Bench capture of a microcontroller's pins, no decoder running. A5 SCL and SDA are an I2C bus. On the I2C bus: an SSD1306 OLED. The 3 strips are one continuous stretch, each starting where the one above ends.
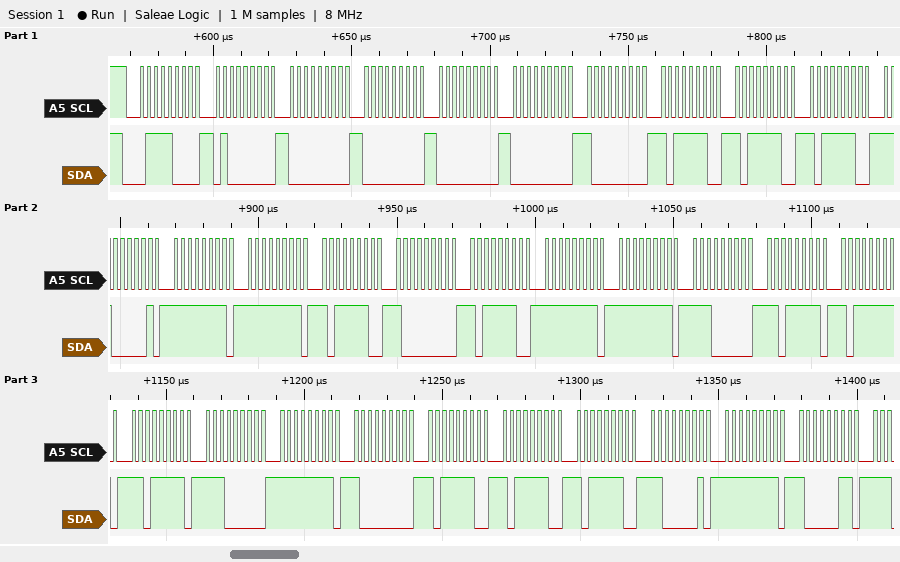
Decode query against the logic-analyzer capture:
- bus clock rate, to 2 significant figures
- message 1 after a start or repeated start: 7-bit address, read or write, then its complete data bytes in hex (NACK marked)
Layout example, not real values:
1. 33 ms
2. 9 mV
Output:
1. 400 kHz
2. 0x3C write: 40 00 00 00 00 80 BE BE BE C1 FF FF BE 80 BE FF FF E0 DF BF DF E0 FF 80 BE BE BE C1 FF 83
